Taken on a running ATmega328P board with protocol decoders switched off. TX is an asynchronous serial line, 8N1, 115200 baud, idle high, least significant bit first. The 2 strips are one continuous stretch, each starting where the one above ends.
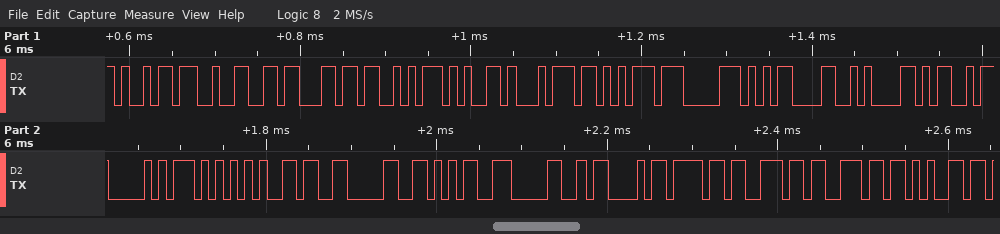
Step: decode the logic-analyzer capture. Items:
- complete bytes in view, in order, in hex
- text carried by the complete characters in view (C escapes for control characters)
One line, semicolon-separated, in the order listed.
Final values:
69 32 63 53 65 74 75 70 0D 0A 4D 50 55 36 30 35 30 43 6F 6E 6E 65; "i2cSetup\r\nMPU6050Conne"
